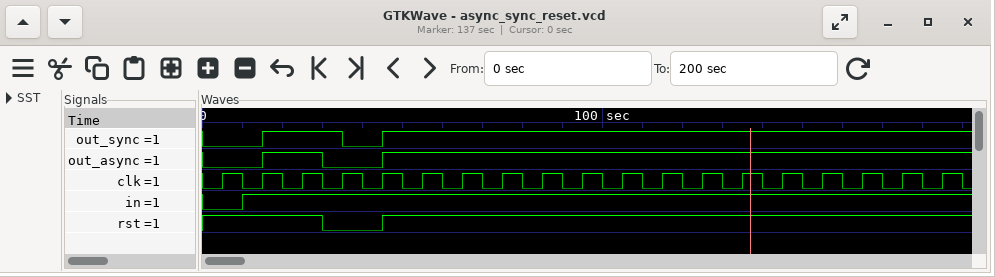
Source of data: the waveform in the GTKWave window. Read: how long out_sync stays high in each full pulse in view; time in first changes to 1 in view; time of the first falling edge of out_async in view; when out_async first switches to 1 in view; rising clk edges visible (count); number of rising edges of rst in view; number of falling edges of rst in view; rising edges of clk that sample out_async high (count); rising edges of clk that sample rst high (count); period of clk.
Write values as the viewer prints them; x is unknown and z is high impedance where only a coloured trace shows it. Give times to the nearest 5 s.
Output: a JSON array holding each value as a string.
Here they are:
["20 s", "10 s", "30 s", "15 s", "19", "1", "1", "15", "17", "10 s"]
